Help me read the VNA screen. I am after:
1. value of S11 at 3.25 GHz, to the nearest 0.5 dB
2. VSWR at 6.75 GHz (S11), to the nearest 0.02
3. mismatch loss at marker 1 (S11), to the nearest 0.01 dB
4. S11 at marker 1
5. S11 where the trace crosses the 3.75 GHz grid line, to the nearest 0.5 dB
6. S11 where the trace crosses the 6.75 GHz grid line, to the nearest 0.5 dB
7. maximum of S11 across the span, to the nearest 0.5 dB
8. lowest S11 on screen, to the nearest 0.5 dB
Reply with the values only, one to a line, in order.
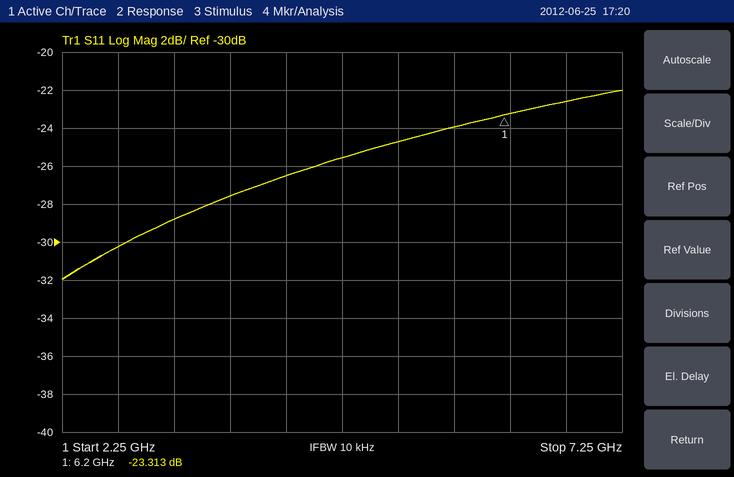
-29.0 dB
1.16
0.02 dB
-23.313 dB
-27.5 dB
-22.5 dB
-22.0 dB
-32.0 dB
